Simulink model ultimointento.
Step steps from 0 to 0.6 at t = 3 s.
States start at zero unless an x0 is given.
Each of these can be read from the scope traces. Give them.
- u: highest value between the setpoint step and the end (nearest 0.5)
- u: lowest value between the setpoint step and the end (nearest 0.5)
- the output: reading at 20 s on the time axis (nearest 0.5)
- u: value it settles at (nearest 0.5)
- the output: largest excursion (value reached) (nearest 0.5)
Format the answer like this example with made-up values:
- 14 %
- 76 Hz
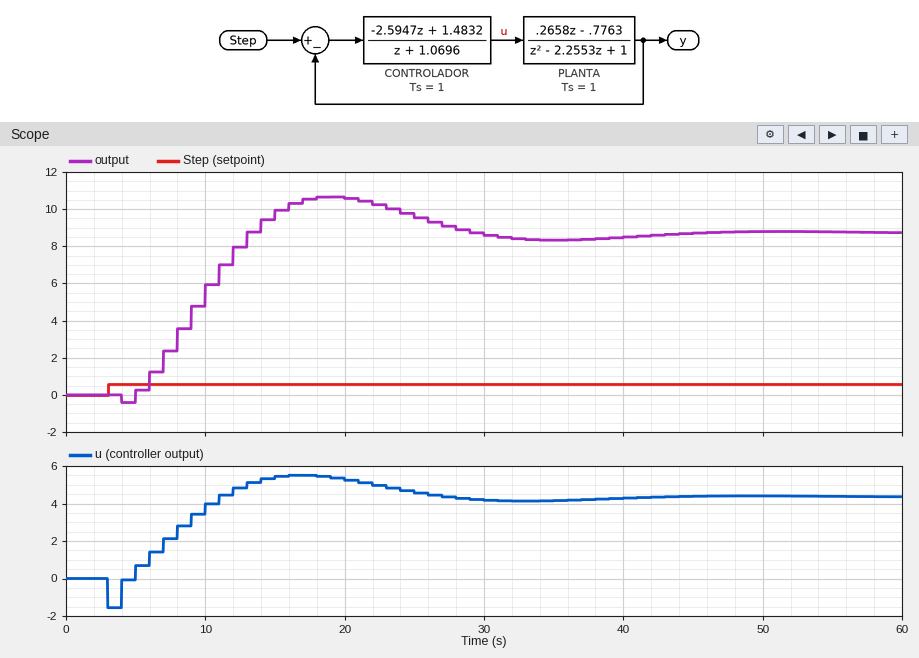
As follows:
- 5.5
- -1.5
- 10.5
- 4.5
- 10.5
